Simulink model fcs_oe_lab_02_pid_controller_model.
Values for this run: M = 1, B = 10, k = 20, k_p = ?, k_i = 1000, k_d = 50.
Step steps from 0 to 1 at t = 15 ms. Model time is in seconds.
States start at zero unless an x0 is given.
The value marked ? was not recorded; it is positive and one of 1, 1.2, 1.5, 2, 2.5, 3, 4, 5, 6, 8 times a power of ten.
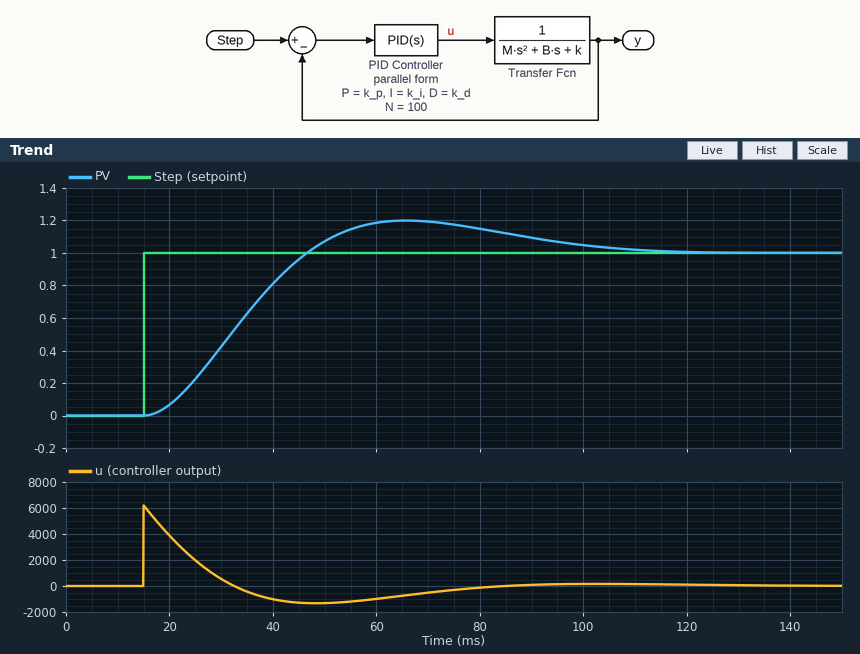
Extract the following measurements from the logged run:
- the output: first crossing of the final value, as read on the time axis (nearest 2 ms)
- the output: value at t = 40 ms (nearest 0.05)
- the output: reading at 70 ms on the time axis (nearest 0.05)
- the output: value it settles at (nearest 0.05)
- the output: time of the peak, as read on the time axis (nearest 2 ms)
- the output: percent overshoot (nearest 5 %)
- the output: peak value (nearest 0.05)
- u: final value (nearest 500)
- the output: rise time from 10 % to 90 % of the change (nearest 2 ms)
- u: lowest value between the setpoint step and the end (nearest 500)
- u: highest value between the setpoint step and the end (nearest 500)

46 ms
0.80
1.20
1.00
66 ms
20 %
1.20
0
22 ms
-1500
6000
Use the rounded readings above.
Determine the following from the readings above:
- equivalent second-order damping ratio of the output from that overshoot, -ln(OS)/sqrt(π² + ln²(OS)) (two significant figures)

0.46
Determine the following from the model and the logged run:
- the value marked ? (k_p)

1200
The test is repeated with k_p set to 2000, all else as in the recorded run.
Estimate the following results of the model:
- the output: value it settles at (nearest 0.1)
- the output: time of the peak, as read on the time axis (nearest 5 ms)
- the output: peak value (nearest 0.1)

1.0
60 ms
1.3
